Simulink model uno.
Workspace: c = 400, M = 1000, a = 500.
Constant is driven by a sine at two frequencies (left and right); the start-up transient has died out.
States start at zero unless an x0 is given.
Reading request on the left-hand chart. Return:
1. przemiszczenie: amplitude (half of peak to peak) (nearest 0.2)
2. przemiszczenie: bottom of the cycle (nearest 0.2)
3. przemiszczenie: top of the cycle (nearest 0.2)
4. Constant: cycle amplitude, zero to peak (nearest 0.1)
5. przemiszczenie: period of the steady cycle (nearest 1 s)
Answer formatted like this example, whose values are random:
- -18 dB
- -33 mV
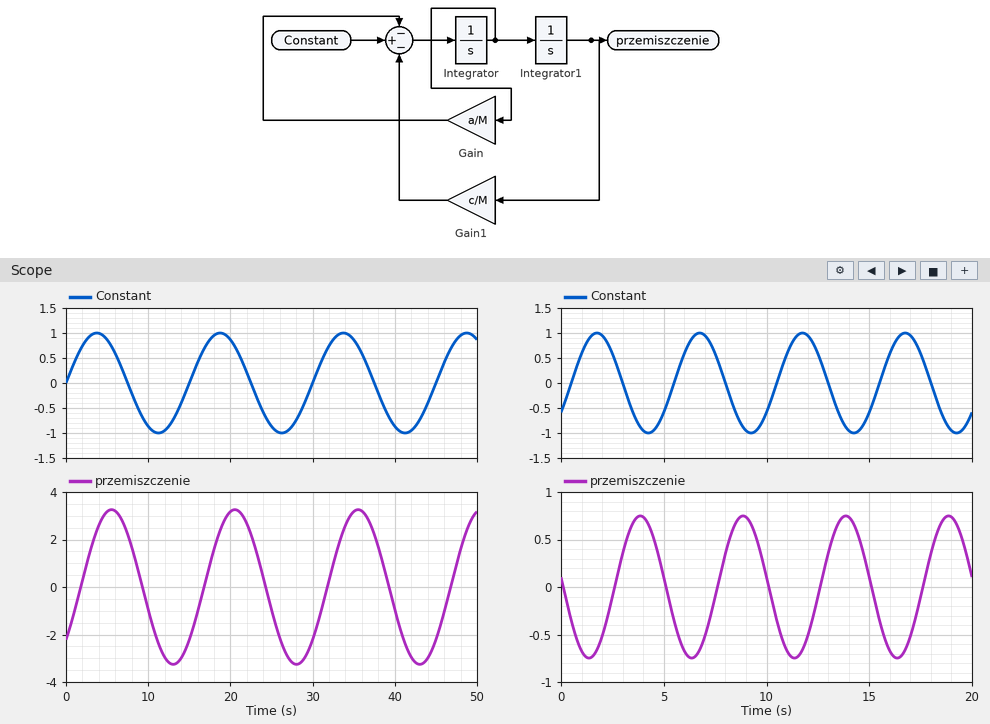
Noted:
- 3.2
- -3.2
- 3.2
- 1.0
- 15 s
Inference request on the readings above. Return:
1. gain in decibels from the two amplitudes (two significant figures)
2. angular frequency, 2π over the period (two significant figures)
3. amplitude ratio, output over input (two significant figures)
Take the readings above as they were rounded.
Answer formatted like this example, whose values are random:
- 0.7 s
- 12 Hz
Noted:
- 10 dB
- 0.42 rad/s
- 3.2
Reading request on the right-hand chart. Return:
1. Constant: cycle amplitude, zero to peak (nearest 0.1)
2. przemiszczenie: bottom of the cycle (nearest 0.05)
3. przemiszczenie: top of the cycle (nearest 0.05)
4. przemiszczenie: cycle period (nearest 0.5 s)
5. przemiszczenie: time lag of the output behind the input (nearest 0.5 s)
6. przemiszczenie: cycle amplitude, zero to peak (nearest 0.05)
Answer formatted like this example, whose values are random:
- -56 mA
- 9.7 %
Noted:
- 1.0
- -0.75
- 0.75
- 5.0 s
- 2.0 s
- 0.75
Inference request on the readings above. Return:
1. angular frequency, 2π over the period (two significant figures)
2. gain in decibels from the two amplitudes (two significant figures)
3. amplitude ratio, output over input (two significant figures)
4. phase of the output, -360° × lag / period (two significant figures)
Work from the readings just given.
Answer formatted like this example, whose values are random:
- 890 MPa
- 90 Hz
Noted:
- 1.3 rad/s
- -2.5 dB
- 0.75
- -140°
